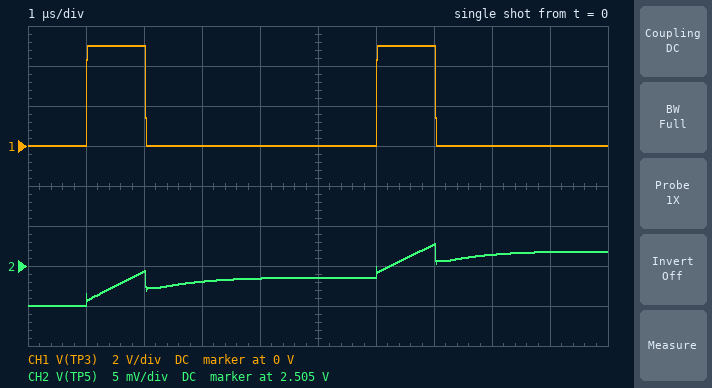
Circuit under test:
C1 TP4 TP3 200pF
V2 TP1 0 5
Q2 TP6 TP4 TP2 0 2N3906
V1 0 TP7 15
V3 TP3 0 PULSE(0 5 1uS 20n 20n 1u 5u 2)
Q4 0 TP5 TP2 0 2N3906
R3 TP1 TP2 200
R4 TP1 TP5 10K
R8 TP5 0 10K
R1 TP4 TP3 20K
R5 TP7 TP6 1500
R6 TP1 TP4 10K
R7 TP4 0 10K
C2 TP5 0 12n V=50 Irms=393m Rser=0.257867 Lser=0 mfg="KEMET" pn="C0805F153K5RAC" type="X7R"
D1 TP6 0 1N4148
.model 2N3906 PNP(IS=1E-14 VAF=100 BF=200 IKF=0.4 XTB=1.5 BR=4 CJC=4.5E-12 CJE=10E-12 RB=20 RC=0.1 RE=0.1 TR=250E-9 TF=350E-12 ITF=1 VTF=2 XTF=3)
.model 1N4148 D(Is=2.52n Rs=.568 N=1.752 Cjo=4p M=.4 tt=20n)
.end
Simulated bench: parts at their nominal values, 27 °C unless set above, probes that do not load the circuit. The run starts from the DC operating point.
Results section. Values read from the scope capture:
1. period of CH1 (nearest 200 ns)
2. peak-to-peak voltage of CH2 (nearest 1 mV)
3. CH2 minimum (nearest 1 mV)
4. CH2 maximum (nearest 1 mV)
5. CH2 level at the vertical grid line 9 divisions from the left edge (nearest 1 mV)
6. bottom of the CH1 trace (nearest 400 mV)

5.0 µs
8 mV
2.500 V
2.508 V
2.507 V
0 V
